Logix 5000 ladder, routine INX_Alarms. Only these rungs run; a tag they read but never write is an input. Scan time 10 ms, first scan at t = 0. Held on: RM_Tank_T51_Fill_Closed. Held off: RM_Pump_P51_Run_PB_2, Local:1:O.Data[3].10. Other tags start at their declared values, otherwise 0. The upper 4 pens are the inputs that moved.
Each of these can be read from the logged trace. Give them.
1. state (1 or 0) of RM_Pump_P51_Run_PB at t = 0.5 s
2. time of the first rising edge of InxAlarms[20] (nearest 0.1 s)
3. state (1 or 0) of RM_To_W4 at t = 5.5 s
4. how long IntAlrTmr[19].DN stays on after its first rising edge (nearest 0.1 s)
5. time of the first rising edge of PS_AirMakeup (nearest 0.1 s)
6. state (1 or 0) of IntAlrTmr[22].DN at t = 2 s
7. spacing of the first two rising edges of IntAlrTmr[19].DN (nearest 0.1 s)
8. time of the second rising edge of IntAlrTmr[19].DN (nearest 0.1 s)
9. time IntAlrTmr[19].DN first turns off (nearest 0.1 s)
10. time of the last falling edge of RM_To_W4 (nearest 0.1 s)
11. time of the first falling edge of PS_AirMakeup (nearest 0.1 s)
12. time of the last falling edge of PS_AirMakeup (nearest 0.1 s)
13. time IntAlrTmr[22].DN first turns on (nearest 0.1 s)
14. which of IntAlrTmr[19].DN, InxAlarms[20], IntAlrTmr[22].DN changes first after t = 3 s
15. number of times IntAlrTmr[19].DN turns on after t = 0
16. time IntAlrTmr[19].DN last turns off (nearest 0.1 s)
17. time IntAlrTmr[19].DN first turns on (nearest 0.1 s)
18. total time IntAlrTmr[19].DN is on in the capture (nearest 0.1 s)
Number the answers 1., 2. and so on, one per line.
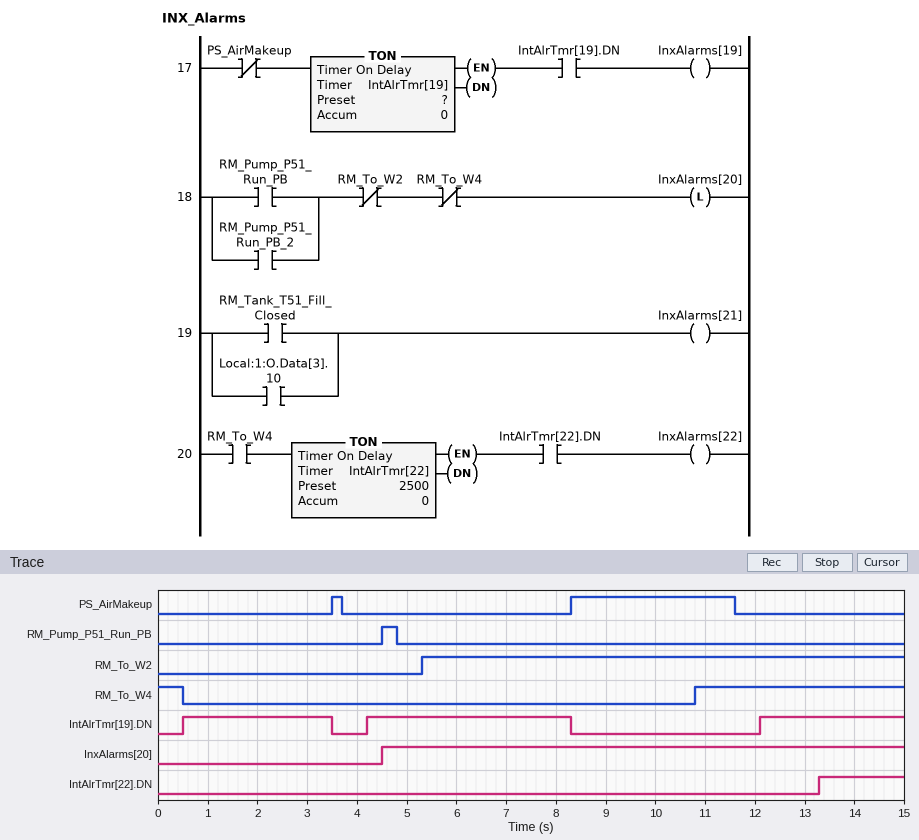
1. 0
2. 4.5 s
3. 0
4. 3.0 s
5. 3.5 s
6. 0
7. 3.7 s
8. 4.2 s
9. 3.5 s
10. 0.5 s
11. 3.7 s
12. 11.6 s
13. 13.3 s
14. IntAlrTmr[19].DN
15. 3
16. 8.3 s
17. 0.5 s
18. 10.0 s
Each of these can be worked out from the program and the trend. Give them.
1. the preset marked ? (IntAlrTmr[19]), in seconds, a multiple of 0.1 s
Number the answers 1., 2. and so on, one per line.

1. 0.5 s
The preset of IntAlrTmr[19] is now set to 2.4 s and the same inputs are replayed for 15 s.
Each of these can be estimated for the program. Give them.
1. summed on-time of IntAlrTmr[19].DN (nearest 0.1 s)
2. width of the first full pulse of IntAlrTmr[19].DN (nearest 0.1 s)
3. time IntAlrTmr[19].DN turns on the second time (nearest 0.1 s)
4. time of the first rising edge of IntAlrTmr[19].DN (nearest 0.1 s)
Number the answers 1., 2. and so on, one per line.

1. 4.3 s
2. 1.1 s
3. 6.1 s
4. 2.4 s
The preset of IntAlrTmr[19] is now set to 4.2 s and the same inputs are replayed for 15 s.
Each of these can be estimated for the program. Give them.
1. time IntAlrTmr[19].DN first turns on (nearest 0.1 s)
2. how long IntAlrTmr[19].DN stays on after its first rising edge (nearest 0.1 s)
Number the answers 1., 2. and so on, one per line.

1. 7.9 s
2. 0.4 s
